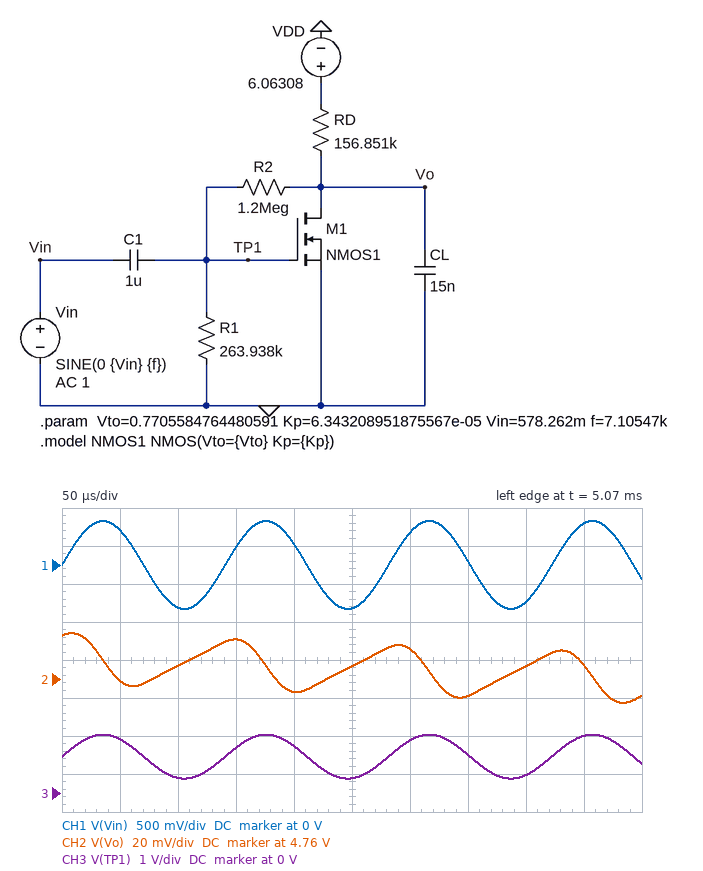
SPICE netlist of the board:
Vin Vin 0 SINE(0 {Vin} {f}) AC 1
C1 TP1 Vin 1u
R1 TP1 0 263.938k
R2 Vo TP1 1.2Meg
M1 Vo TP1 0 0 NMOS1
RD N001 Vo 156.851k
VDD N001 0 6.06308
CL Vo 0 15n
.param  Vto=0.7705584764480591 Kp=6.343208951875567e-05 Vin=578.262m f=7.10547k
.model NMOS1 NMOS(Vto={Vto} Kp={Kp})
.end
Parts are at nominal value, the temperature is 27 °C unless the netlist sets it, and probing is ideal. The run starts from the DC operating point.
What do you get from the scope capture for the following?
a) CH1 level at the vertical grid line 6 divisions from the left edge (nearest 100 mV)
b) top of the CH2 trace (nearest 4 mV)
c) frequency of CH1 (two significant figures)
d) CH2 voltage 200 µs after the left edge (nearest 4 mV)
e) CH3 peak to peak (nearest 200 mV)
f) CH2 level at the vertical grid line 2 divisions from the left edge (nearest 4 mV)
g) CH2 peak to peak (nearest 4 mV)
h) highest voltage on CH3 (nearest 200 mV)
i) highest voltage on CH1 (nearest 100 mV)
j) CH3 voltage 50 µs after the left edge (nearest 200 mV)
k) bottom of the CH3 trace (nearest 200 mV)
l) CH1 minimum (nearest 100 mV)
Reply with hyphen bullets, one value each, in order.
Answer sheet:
- 400 mV
- 4.784 V
- 7.1 kHz
- 4.752 V
- 1.2 V
- 4.768 V
- 36 mV
- 1.6 V
- 600 mV
- 1.4 V
- 400 mV
- -600 mV
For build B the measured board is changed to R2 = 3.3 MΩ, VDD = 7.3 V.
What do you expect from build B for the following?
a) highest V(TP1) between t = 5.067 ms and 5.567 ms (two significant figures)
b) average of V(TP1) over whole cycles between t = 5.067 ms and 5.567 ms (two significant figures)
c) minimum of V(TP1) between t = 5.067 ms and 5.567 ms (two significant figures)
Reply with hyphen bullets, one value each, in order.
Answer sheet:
- 1.1 V
- 520 mV
- -61 mV
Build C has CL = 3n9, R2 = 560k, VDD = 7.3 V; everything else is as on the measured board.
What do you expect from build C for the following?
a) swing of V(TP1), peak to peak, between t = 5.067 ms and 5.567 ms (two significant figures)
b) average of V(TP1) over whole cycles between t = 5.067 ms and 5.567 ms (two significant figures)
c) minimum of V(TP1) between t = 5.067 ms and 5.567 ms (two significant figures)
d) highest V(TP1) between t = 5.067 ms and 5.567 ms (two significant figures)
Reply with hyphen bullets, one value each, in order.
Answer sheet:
- 1.2 V
- 1.4 V
- 830 mV
- 2.0 V
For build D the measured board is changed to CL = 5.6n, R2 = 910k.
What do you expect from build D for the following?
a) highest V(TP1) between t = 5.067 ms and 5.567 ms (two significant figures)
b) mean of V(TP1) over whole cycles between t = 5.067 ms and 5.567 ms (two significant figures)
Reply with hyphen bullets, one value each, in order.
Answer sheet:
- 1.7 V
- 1.1 V
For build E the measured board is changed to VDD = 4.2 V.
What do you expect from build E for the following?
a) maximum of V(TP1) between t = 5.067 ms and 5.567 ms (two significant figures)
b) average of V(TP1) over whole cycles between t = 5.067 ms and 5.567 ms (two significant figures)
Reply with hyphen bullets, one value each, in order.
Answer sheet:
- 1.3 V
- 680 mV
